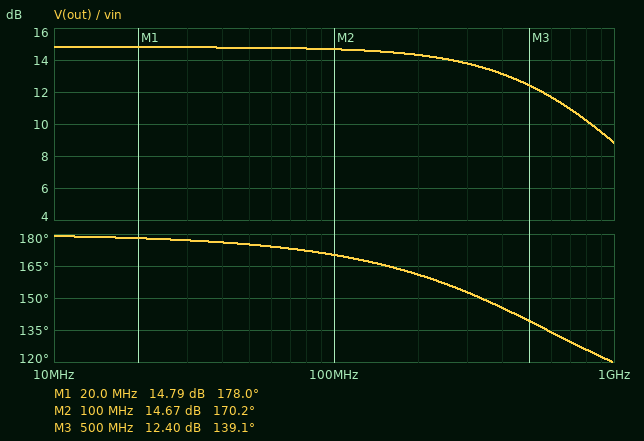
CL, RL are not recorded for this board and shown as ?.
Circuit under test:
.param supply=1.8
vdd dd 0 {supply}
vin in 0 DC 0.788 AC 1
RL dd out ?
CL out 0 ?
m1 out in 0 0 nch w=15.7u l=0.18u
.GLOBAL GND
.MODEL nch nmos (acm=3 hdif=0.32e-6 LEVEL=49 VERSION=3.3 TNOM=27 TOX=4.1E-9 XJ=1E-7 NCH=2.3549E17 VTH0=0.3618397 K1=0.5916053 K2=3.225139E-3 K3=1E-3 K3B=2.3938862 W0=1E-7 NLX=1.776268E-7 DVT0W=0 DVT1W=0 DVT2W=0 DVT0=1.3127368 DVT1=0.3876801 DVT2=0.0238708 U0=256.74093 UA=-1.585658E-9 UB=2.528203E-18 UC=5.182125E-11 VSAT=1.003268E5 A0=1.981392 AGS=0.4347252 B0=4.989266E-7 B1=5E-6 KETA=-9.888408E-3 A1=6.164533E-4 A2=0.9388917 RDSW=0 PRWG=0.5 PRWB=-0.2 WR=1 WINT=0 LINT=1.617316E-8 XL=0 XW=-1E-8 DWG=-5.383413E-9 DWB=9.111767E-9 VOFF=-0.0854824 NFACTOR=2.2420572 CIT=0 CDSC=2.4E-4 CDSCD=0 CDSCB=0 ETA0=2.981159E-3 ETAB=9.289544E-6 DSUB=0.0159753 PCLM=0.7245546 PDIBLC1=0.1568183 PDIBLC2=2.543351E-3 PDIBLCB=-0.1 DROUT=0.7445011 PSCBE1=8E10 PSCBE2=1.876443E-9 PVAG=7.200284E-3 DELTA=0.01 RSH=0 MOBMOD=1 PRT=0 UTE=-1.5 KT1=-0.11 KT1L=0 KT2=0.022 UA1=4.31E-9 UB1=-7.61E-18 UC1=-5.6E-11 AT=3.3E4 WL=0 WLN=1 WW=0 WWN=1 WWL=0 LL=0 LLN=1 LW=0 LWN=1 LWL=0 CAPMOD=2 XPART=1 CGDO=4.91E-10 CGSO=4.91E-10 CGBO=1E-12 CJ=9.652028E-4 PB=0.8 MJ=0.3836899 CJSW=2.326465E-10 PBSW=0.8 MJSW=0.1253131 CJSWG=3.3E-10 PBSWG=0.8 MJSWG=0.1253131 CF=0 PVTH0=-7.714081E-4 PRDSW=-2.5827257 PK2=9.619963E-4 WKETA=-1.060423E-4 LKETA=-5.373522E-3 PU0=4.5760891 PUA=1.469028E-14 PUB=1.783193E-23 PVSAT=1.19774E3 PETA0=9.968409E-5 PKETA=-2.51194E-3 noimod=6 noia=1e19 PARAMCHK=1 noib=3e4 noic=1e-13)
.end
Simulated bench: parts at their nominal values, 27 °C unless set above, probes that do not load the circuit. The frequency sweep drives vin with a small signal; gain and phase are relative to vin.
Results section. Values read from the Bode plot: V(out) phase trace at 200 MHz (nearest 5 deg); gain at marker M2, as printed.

160 deg
14.67 dB
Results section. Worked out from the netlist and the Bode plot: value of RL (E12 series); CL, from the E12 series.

1.2 kΩ
270 fF
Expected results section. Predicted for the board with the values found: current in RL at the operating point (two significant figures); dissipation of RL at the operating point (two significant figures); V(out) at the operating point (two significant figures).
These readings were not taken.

1.0 mA
1.3 mW
560 mV
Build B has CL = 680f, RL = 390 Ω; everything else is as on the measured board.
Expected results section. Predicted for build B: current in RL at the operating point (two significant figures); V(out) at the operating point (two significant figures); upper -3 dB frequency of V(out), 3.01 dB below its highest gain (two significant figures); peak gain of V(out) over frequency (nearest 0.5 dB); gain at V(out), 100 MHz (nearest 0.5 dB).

1.2 mA
1.3 V
630 MHz
7.5 dB
7.0 dB
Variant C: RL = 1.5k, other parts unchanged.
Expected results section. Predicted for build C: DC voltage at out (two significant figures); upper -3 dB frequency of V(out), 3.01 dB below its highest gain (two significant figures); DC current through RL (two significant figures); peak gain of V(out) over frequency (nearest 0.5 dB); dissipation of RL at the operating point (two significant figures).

350 mV
570 MHz
970 µA
14.5 dB
1.4 mW
